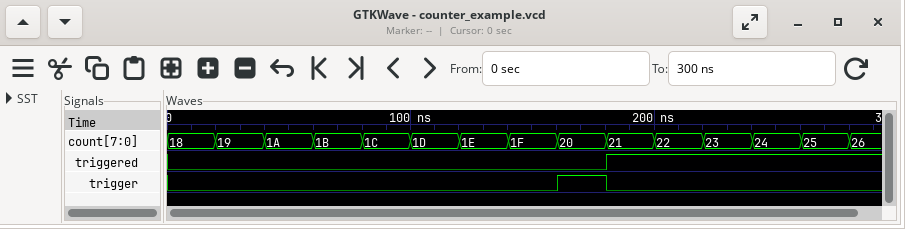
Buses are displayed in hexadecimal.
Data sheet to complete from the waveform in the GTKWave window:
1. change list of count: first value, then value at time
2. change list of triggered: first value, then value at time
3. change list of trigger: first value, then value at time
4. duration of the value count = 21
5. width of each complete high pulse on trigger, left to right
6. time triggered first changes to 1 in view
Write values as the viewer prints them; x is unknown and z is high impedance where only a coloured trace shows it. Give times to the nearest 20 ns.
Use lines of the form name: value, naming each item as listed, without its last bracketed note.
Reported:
change list of count: first value, then value at time: 18, 19 at 20 ns, 1A at 40 ns, 1B at 60 ns, 1C at 80 ns, 1D at 100 ns, 1E at 120 ns, 1F at 140 ns, 20 at 160 ns, 21 at 180 ns, 22 at 200 ns, 23 at 220 ns, 24 at 240 ns, 25 at 260 ns, 26 at 280 ns
change list of triggered: first value, then value at time: 0, 1 at 180 ns
change list of trigger: first value, then value at time: 0, 1 at 160 ns, 0 at 180 ns
duration of the value count = 21: 20 ns
width of each complete high pulse on trigger, left to right: 20 ns
time triggered first changes to 1 in view: 180 ns
